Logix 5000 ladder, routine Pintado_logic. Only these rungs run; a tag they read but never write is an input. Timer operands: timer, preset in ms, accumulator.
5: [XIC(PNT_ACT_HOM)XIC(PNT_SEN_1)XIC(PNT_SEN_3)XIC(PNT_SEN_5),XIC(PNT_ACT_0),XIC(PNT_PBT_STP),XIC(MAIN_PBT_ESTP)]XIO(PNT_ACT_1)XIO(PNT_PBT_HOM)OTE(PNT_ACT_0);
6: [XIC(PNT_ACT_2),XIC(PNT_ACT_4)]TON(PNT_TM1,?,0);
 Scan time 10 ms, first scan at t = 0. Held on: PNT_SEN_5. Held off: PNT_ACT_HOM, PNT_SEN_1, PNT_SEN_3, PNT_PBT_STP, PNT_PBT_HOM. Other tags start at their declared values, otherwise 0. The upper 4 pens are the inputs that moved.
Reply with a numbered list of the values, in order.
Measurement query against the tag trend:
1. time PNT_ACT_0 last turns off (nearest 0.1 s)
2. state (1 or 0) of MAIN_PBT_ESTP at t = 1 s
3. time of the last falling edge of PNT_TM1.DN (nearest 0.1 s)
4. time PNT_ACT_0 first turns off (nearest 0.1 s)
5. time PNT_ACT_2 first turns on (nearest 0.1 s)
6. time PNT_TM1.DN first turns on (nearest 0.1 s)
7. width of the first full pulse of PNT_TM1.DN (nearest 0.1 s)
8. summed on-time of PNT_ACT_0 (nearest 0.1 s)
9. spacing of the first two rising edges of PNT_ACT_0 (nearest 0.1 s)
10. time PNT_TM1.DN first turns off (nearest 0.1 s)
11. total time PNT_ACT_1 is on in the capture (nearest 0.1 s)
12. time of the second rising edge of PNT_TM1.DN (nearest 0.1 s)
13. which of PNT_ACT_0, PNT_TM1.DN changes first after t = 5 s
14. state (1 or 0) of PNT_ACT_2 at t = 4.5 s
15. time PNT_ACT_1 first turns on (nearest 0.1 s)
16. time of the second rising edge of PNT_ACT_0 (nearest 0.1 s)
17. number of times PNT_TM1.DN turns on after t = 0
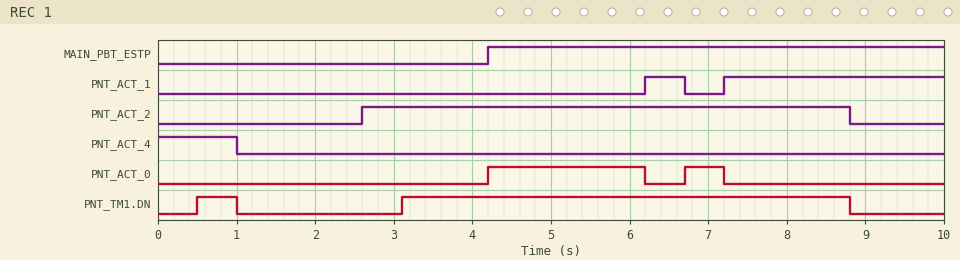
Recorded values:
1. 7.2 s
2. 0
3. 8.8 s
4. 6.2 s
5. 2.6 s
6. 0.5 s
7. 0.5 s
8. 2.5 s
9. 2.5 s
10. 1.0 s
11. 3.3 s
12. 3.1 s
13. PNT_ACT_0
14. 1
15. 6.2 s
16. 6.7 s
17. 2
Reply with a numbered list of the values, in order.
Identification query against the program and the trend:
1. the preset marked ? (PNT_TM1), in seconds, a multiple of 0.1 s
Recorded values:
1. 0.5 s
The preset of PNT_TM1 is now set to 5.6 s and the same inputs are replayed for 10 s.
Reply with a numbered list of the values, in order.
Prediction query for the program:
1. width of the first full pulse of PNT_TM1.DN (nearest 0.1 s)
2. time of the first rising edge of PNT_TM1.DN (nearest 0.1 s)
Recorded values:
1. 0.6 s
2. 8.2 s
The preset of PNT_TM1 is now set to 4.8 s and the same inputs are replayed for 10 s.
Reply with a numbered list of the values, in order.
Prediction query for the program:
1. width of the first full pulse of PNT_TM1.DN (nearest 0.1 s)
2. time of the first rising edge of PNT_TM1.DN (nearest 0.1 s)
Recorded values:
1. 1.4 s
2. 7.4 s
